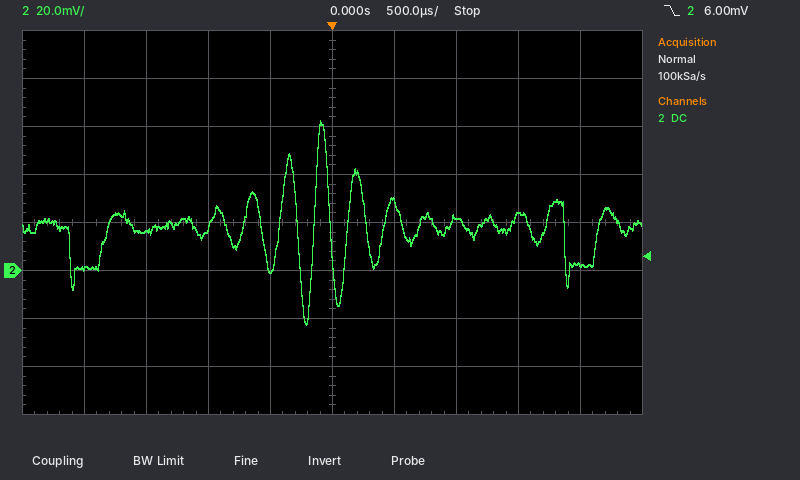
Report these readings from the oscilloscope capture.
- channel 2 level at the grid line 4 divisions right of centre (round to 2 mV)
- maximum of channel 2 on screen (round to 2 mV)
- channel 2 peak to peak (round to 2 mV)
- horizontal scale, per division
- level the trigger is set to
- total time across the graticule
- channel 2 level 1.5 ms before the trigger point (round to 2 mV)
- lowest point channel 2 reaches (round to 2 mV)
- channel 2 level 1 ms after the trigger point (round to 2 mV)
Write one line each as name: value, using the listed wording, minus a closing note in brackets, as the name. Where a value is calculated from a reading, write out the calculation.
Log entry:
channel 2 level at the grid line 4 divisions right of centre: 2 mV
maximum of channel 2 on screen: 62 mV
channel 2 peak to peak: 62 mV − (-22 mV) = 84 mV
horizontal scale, per division: 500 µs
level the trigger is set to: 6.00 mV
total time across the graticule: 5 ms
channel 2 level 1.5 ms before the trigger point: 16 mV
lowest point channel 2 reaches: -22 mV
channel 2 level 1 ms after the trigger point: 22 mV
